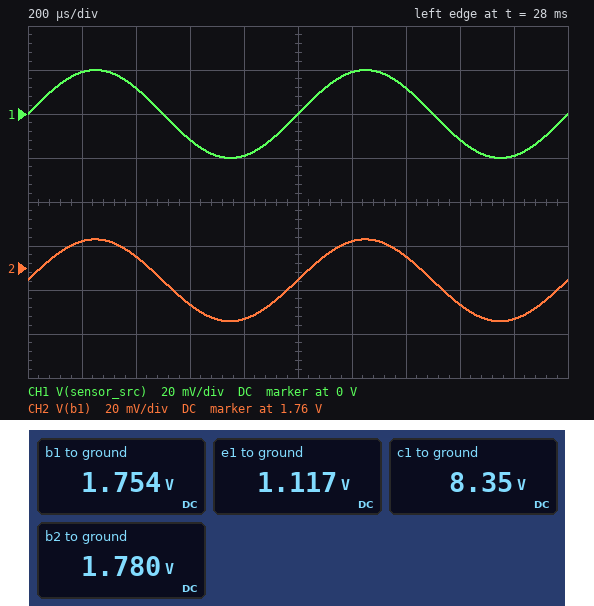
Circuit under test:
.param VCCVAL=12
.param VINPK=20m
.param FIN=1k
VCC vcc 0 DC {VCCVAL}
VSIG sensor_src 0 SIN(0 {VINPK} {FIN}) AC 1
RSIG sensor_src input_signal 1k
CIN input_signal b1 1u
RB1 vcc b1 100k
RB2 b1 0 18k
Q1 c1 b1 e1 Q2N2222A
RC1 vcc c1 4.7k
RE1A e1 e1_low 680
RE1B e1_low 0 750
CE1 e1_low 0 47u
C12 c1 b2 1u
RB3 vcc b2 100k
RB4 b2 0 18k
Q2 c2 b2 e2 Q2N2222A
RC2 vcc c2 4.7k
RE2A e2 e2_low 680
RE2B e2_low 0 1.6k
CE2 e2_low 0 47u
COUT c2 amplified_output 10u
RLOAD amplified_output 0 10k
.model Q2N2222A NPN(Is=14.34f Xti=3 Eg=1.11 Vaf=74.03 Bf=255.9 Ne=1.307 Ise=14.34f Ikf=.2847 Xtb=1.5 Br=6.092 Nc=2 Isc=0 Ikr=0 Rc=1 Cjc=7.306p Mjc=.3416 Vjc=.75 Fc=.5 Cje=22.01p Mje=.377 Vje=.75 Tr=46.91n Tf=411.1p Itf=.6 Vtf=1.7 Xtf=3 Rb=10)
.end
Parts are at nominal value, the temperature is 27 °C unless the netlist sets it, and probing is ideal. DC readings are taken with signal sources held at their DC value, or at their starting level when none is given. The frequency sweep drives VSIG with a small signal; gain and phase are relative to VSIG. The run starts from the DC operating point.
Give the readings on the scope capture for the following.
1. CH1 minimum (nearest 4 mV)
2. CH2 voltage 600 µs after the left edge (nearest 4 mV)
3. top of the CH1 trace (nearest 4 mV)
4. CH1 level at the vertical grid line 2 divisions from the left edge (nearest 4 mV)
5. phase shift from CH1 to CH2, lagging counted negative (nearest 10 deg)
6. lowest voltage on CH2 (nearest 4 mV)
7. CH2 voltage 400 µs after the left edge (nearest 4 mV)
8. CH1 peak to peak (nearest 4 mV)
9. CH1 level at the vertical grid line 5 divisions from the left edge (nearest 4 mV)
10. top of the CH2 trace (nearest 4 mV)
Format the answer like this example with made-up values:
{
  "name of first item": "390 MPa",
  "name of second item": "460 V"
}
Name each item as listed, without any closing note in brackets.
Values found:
{
  "CH1 minimum": "-20 mV",
  "CH2 voltage 600 µs after the left edge": "1.744 V",
  "top of the CH1 trace": "20 mV",
  "CH1 level at the vertical grid line 2 divisions from the left edge": "12 mV",
  "phase shift from CH1 to CH2, lagging counted negative": "0 deg",
  "lowest voltage on CH2": "1.736 V",
  "CH2 voltage 400 µs after the left edge": "1.764 V",
  "CH1 peak to peak": "40 mV",
  "CH1 level at the vertical grid line 5 divisions from the left edge": "0 V",
  "top of the CH2 trace": "1.772 V"
}
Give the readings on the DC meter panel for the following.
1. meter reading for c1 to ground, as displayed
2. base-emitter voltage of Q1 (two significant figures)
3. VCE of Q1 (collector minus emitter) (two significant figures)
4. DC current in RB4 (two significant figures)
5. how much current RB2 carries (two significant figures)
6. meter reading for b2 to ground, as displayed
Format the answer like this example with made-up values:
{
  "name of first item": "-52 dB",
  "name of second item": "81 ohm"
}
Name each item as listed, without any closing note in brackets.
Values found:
{
  "meter reading for c1 to ground, as displayed": "8.35 V",
  "base-emitter voltage of Q1": "640 mV",
  "VCE of Q1 (collector minus emitter)": "7.2 V",
  "DC current in RB4": "99 µA",
  "how much current RB2 carries": "97 µA",
  "meter reading for b2 to ground, as displayed": "1.780 V"
}
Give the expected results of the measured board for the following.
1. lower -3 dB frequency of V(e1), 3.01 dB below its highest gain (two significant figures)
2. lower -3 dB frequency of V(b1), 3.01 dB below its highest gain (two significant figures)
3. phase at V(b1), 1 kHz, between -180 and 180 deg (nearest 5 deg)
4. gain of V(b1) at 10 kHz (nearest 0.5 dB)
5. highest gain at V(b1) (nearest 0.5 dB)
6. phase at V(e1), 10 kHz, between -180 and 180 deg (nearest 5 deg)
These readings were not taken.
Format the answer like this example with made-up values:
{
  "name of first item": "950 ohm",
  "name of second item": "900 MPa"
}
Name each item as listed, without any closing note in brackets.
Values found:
{
  "lower -3 dB frequency of V(e1), 3.01 dB below its highest gain": "11 Hz",
  "lower -3 dB frequency of V(b1), 3.01 dB below its highest gain": "11 Hz",
  "phase at V(b1), 1 kHz, between -180 and 180 deg": "0 deg",
  "gain of V(b1) at 10 kHz": "-0.5 dB",
  "highest gain at V(b1)": "-0.5 dB",
  "phase at V(e1), 10 kHz, between -180 and 180 deg": "0 deg"
}
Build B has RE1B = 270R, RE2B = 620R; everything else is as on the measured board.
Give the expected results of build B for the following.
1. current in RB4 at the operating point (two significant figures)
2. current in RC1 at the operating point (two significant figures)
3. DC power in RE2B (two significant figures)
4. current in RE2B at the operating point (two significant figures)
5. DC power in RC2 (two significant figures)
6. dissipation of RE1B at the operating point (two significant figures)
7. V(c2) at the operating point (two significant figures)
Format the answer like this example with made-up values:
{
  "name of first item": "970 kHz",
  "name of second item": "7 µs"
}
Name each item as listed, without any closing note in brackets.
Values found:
{
  "current in RB4 at the operating point": "97 µA",
  "current in RC1 at the operating point": "1.1 mA",
  "DC power in RE2B": "450 µW",
  "current in RE2B at the operating point": "850 µA",
  "DC power in RC2": "3.4 mW",
  "dissipation of RE1B at the operating point": "350 µW",
  "V(c2) at the operating point": "8.0 V"
}
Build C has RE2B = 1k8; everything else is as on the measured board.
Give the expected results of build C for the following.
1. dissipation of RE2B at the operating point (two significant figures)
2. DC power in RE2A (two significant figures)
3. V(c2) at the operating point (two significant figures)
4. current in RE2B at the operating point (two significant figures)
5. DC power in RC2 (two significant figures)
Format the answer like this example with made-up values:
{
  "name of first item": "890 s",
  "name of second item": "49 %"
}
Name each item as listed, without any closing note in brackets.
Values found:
{
  "dissipation of RE2B at the operating point": "390 µW",
  "DC power in RE2A": "150 µW",
  "V(c2) at the operating point": "9.8 V",
  "current in RE2B at the operating point": "470 µA",
  "DC power in RC2": "1.0 mW"
}
